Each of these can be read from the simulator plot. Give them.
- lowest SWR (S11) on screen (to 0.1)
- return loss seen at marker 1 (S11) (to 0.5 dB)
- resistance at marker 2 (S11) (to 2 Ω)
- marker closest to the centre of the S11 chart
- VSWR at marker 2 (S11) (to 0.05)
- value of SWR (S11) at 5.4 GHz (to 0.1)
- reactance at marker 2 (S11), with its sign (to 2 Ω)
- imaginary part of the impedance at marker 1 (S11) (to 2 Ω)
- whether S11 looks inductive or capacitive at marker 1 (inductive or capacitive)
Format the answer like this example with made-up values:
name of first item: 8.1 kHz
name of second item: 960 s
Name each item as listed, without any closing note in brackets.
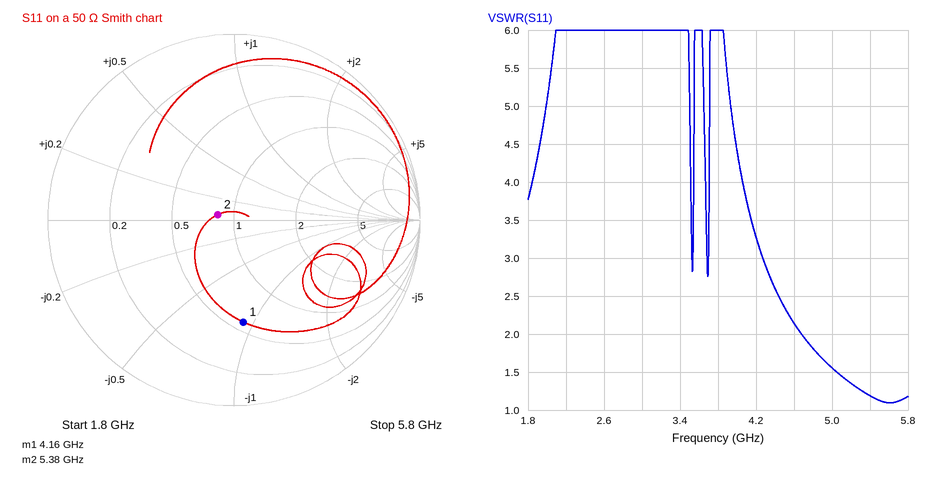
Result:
lowest SWR (S11) on screen: 1.1
return loss seen at marker 1 (S11): 5.0 dB
resistance at marker 2 (S11): 42 Ω
marker closest to the centre of the S11 chart: marker 2
VSWR at marker 2 (S11): 1.20
value of SWR (S11) at 5.4 GHz: 1.2
reactance at marker 2 (S11), with its sign: +2 Ω
imaginary part of the impedance at marker 1 (S11): -46 Ω
whether S11 looks inductive or capacitive at marker 1: capacitive
